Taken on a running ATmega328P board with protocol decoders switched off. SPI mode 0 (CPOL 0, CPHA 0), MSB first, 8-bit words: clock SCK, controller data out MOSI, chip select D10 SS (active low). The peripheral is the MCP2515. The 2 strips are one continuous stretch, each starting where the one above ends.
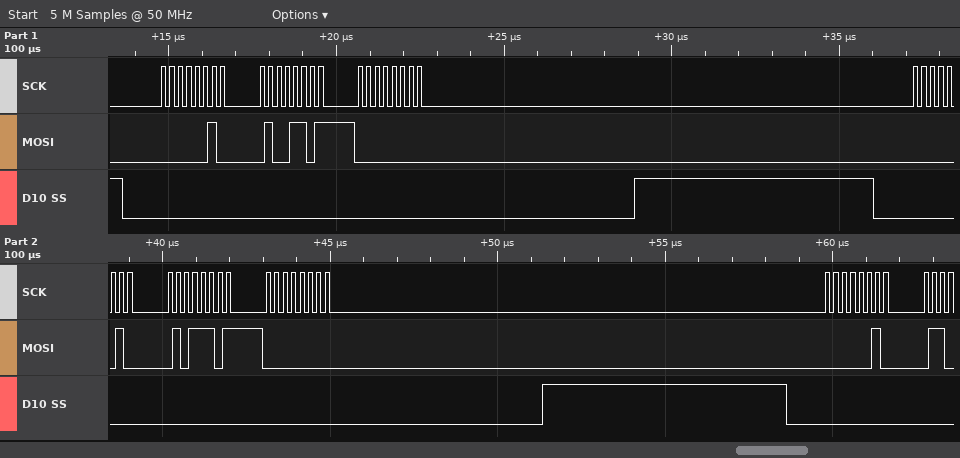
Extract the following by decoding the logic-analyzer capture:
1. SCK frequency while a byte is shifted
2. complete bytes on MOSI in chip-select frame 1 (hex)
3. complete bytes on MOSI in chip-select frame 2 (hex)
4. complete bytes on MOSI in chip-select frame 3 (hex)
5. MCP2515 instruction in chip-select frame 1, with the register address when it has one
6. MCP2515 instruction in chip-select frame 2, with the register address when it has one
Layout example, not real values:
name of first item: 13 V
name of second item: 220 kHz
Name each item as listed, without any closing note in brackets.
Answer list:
SCK frequency while a byte is shifted: 4 MHz
complete bytes on MOSI in chip-select frame 1: 02 4D 00
complete bytes on MOSI in chip-select frame 2: 02 5D 00
complete bytes on MOSI in chip-select frame 3: 02
MCP2515 instruction in chip-select frame 1, with the register address when it has one: WRITE 0x4D
MCP2515 instruction in chip-select frame 2, with the register address when it has one: WRITE 0x5D
